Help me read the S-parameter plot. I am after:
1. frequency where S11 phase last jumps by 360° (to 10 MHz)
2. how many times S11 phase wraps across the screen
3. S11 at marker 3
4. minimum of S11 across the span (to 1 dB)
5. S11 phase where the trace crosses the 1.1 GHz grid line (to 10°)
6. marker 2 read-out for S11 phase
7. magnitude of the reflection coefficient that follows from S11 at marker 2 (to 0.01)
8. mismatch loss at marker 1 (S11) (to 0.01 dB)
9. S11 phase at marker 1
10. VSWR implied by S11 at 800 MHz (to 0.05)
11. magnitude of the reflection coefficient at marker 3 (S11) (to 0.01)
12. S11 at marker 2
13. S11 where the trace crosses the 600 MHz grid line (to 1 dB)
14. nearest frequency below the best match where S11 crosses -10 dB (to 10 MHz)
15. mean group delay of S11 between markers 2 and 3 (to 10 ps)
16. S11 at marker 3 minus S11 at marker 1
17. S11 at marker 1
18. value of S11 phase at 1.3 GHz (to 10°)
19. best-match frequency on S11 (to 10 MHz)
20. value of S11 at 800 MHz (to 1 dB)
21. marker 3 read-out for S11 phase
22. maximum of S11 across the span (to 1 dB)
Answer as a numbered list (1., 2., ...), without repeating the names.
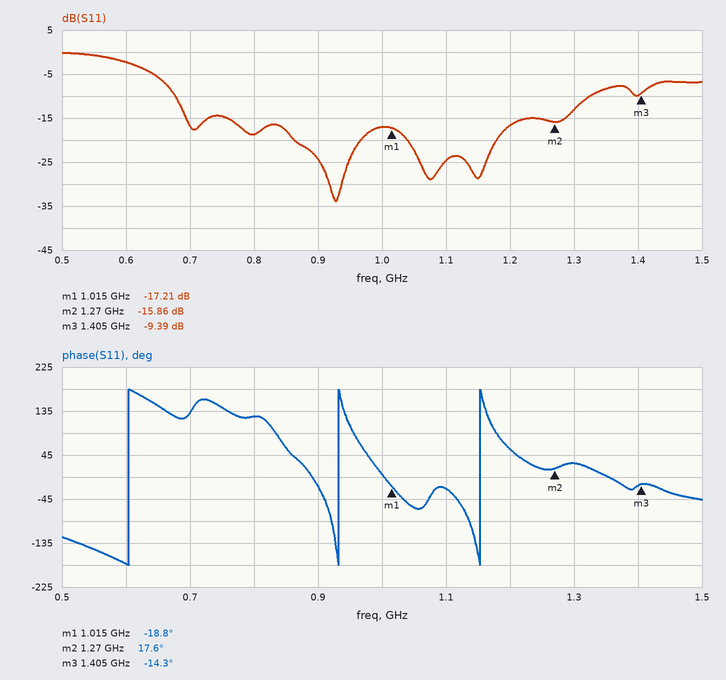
1. 1.15 GHz
2. 3
3. -9.39 dB
4. -34 dB
5. -20°
6. 17.6°
7. 0.16
8. 0.08 dB
9. -18.8°
10. 1.25
11. 0.34
12. -15.86 dB
13. -2 dB
14. 680 MHz
15. 660 ps
16. 7.82 dB
17. -17.21 dB
18. 30°
19. 930 MHz
20. -19 dB
21. -14.3°
22. 0 dB
